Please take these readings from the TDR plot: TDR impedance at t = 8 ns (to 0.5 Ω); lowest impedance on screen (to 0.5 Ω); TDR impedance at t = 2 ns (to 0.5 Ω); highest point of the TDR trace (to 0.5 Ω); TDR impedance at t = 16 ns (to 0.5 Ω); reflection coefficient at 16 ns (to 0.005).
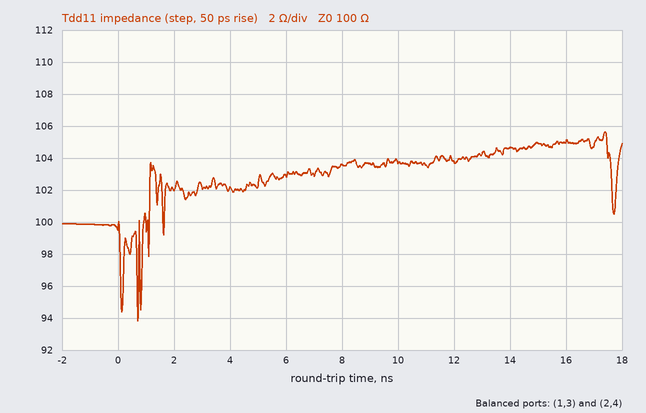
103.5 Ω
94.0 Ω
102.0 Ω
105.5 Ω
105.0 Ω
+0.025
